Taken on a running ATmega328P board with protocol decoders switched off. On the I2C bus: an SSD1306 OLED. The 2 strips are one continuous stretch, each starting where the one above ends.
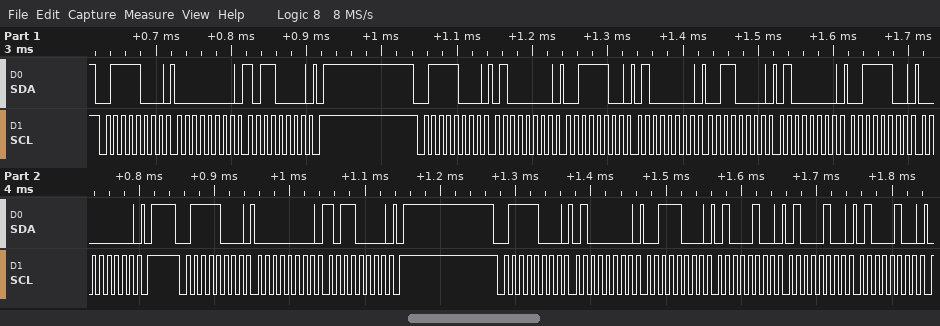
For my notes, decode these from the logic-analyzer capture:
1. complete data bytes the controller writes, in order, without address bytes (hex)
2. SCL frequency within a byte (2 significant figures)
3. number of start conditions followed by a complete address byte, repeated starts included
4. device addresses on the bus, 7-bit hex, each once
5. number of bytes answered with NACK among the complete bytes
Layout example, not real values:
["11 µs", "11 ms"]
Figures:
["00 B0 40 3C 40 30 40 3C 00 00 B0 40 38 44 44 44", "100 kHz", "4", "0x3C", "0"]
